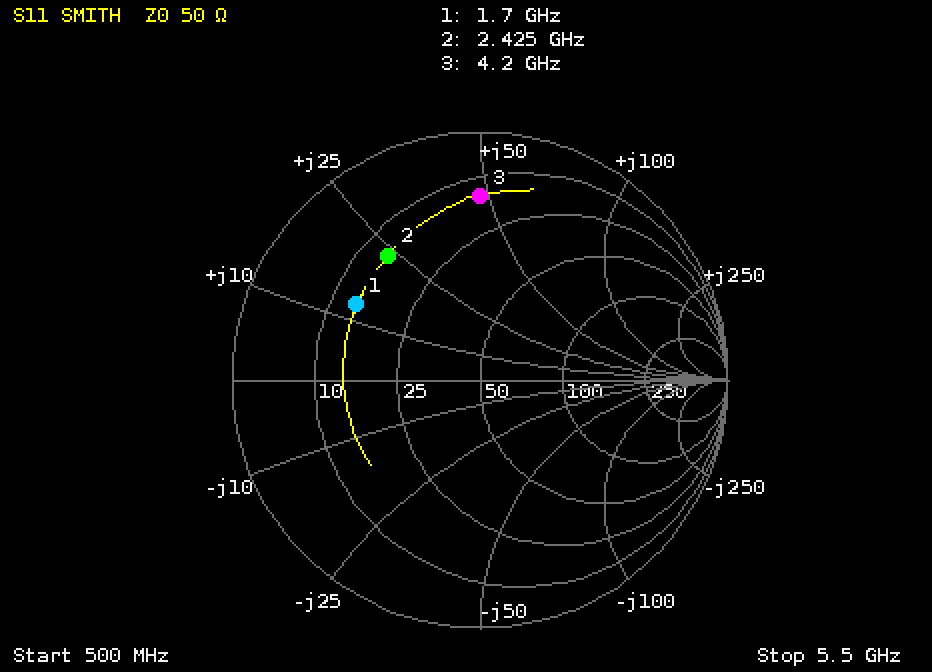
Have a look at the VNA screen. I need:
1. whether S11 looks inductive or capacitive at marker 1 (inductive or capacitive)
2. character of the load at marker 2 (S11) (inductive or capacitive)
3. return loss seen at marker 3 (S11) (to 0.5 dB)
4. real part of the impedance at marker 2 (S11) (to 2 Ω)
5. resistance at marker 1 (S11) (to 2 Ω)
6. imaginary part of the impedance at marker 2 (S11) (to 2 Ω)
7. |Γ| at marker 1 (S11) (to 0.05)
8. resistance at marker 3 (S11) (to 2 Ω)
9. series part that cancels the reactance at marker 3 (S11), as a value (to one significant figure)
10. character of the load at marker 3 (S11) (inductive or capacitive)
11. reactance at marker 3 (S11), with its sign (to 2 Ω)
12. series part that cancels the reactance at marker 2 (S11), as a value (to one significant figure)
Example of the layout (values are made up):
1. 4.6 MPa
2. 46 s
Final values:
1. inductive
2. inductive
3. 2.5 dB
4. 14 Ω
5. 14 Ω
6. +24 Ω
7. 0.60
8. 14 Ω
9. 800 fF
10. inductive
11. +48 Ω
12. 3 pF
